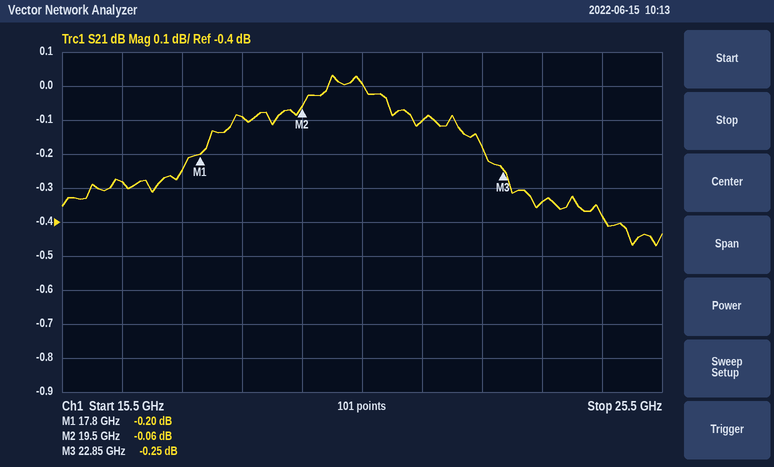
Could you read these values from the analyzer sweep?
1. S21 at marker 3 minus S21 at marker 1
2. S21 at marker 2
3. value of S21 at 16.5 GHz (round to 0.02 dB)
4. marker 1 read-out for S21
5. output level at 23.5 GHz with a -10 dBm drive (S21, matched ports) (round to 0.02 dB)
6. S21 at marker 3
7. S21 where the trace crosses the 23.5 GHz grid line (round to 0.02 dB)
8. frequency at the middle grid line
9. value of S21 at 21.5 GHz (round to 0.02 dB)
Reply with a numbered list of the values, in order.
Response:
1. -0.05 dB
2. -0.06 dB
3. -0.28 dB
4. -0.20 dB
5. -10.34 dBm
6. -0.25 dB
7. -0.34 dB
8. 20.5 GHz
9. -0.10 dB
